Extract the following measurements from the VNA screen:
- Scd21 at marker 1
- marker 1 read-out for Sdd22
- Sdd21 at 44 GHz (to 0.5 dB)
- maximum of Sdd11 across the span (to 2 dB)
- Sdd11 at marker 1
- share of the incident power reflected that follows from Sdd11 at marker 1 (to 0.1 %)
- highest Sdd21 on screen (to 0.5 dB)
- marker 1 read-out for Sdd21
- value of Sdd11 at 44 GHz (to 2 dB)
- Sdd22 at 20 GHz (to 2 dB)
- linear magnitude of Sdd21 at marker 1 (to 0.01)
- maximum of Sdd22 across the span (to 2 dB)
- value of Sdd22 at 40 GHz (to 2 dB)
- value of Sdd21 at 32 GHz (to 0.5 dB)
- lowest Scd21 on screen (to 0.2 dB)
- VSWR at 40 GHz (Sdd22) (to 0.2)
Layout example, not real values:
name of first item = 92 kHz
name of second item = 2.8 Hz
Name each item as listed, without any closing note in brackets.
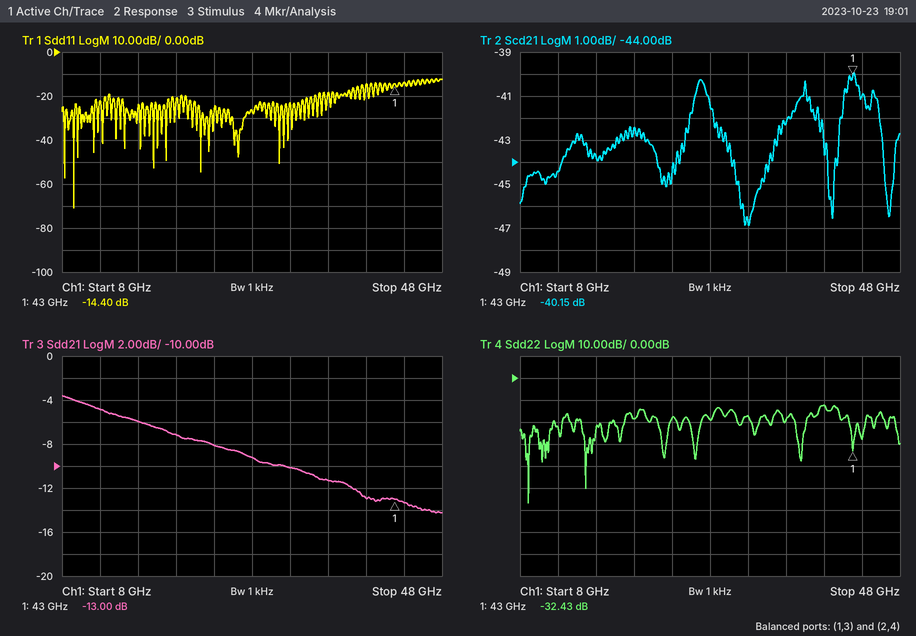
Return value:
Scd21 at marker 1 = -40.15 dB
marker 1 read-out for Sdd22 = -32.43 dB
Sdd21 at 44 GHz = -13.5 dB
maximum of Sdd11 across the span = -12 dB
Sdd11 at marker 1 = -14.40 dB
share of the incident power reflected that follows from Sdd11 at marker 1 = 3.6 %
highest Sdd21 on screen = -3.5 dB
marker 1 read-out for Sdd21 = -13.00 dB
value of Sdd11 at 44 GHz = -14 dB
Sdd22 at 20 GHz = -18 dB
linear magnitude of Sdd21 at marker 1 = 0.22
maximum of Sdd22 across the span = -12 dB
value of Sdd22 at 40 GHz = -12 dB
value of Sdd21 at 32 GHz = -10.0 dB
lowest Scd21 on screen = -46.8 dB
VSWR at 40 GHz (Sdd22) = 1.6
